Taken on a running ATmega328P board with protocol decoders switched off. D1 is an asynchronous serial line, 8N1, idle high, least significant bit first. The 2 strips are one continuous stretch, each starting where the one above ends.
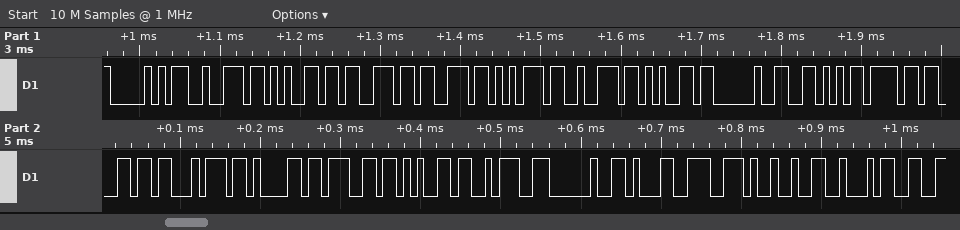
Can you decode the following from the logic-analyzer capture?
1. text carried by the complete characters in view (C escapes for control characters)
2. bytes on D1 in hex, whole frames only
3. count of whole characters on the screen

"Pressure Voltage: 1.24"
50 72 65 73 73 75 72 65 20 56 6F 6C 74 61 67 65 3A 20 31 2E 32 34
22
